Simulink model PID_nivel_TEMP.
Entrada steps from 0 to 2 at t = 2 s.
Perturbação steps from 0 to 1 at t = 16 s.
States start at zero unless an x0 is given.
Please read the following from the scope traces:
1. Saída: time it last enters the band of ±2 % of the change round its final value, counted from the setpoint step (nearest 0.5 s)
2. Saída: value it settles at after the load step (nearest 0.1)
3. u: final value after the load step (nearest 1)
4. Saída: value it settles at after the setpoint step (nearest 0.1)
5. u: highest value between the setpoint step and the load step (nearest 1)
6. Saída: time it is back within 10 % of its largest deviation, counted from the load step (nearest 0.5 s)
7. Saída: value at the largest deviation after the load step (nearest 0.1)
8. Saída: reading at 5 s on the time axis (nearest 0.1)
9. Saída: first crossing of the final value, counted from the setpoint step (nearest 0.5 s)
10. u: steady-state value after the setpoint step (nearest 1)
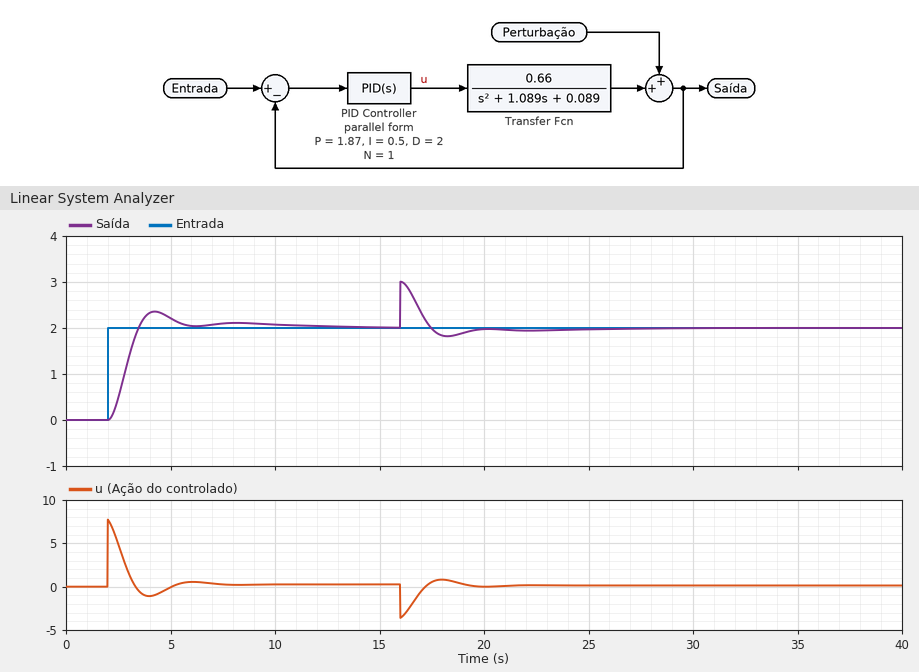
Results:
10.5 s
2.0
0
2.0
8
3.0 s
3.0
2.2
1.5 s
0
